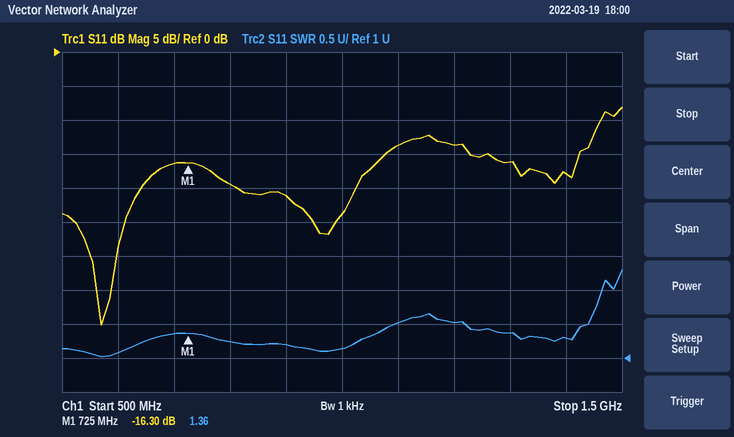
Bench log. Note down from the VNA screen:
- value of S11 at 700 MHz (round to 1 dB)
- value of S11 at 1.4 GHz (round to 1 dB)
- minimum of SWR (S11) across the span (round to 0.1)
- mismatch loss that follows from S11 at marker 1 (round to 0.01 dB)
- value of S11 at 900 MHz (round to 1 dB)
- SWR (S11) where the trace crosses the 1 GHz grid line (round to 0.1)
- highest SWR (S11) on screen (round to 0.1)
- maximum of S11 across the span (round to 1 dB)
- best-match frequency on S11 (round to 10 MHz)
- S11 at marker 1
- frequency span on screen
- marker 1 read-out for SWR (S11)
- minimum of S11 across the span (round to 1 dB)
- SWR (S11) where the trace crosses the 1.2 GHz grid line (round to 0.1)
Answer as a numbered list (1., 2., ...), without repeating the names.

1. -16 dB
2. -18 dB
3. 1.0
4. 0.10 dB
5. -21 dB
6. 1.1
7. 2.3
8. -8 dB
9. 570 MHz
10. -16.30 dB
11. 1 GHz
12. 1.36
13. -40 dB
14. 1.5
